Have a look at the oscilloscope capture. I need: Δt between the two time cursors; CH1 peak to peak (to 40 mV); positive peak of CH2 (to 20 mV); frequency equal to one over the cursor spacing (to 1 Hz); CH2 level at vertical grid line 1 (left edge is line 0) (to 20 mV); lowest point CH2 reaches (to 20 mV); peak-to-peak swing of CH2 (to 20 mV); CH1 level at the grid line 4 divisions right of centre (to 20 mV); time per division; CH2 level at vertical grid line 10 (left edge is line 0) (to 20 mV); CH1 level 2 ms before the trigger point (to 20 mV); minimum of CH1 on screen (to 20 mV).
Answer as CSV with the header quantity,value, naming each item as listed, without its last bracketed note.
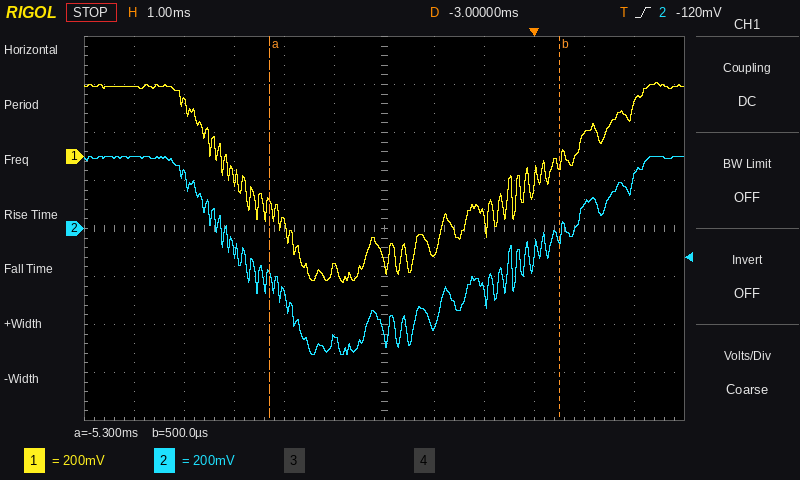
quantity,value
Δt between the two time cursors,5.8 ms
CH1 peak to peak,840 mV
positive peak of CH2,300 mV
frequency equal to one over the cursor spacing,172 Hz
CH2 level at vertical grid line 1 (left edge is line 0),300 mV
lowest point CH2 reaches,-520 mV
peak-to-peak swing of CH2,820 mV
CH1 level at the grid line 4 divisions right of centre,100 mV
time per division,1 ms
CH2 level at vertical grid line 10 (left edge is line 0),100 mV
CH1 level 2 ms before the trigger point,-400 mV
minimum of CH1 on screen,-520 mV
